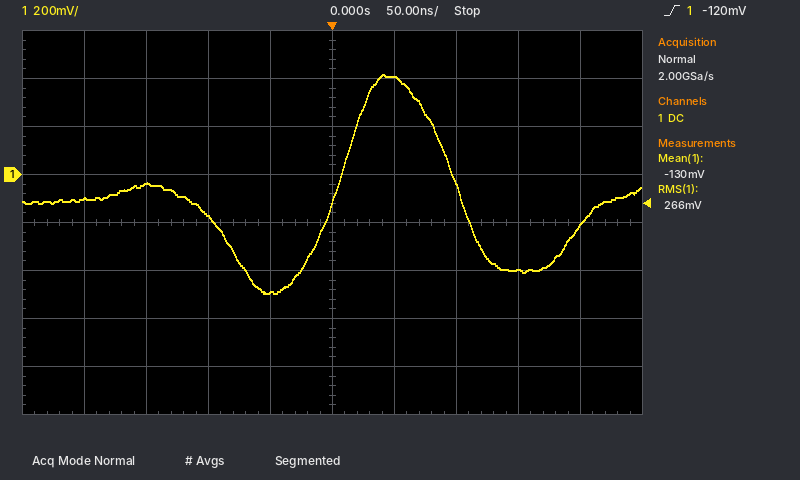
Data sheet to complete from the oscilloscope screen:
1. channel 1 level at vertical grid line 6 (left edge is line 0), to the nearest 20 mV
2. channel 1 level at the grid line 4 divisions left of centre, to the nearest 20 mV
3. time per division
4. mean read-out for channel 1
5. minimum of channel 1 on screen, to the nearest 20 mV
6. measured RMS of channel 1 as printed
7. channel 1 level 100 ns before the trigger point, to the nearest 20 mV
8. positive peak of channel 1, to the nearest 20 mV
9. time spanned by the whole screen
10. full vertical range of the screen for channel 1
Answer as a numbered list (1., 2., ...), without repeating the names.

1. 400 mV
2. -100 mV
3. 50 ns
4. -130 mV
5. -500 mV
6. 266 mV
7. -180 mV
8. 420 mV
9. 500 ns
10. 1.6 V
